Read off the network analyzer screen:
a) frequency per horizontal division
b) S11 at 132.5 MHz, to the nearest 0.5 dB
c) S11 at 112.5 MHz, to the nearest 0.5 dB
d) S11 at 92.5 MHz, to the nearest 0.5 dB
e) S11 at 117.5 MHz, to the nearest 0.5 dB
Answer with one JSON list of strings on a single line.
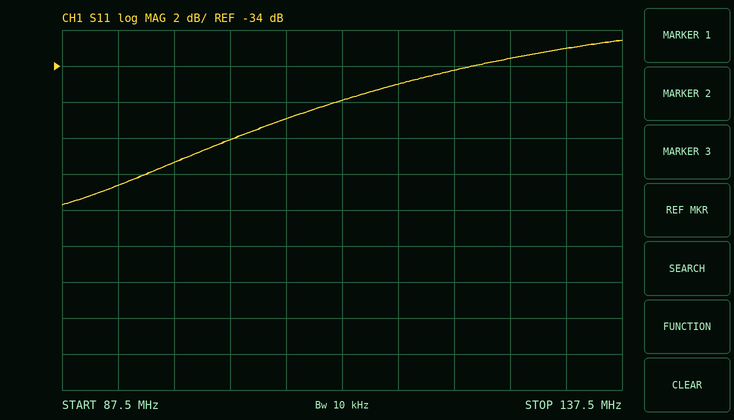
["5 MHz", "-33.0 dB", "-36.0 dB", "-40.5 dB", "-35.0 dB"]
